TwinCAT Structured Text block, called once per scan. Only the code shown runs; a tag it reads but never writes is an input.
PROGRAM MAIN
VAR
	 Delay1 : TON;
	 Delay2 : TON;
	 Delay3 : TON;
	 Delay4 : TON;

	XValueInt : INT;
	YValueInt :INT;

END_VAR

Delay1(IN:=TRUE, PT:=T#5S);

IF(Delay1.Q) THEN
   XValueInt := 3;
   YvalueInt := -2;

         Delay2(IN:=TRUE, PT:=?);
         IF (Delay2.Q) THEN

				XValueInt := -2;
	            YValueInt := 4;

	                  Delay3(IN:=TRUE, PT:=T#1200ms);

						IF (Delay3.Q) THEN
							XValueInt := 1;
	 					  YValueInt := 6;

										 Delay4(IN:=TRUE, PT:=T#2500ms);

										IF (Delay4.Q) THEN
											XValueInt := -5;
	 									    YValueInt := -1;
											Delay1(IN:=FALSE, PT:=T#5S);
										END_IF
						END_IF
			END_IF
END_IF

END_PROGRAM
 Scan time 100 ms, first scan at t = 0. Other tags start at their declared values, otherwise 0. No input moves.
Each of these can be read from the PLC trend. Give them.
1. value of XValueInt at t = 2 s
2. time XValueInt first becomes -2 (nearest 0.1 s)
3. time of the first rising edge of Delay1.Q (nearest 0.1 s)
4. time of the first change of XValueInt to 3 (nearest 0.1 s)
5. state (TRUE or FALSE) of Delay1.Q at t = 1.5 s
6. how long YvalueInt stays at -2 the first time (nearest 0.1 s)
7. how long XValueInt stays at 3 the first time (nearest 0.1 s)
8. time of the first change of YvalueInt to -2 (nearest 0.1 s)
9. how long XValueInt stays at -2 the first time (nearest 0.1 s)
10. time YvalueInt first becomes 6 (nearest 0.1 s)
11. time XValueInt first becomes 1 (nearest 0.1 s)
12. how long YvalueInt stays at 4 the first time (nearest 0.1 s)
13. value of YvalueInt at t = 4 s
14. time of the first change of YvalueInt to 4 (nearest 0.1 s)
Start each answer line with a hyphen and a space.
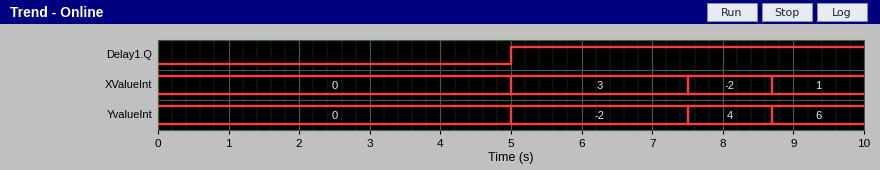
- 0
- 7.5 s
- 5.0 s
- 5.0 s
- FALSE
- 2.5 s
- 2.5 s
- 5.0 s
- 1.2 s
- 8.7 s
- 8.7 s
- 1.2 s
- 0
- 7.5 s
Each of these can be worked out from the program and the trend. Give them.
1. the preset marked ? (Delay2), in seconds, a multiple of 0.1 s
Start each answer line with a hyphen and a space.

- 2.5 s
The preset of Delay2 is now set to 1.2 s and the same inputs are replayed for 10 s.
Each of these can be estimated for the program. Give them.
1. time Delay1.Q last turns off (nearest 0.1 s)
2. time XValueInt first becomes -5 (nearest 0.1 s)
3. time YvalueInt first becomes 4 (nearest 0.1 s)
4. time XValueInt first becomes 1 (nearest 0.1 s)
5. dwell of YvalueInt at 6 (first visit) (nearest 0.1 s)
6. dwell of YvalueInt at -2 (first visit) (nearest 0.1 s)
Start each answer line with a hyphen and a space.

- 9.9 s
- 9.9 s
- 6.2 s
- 7.4 s
- 2.5 s
- 1.2 s
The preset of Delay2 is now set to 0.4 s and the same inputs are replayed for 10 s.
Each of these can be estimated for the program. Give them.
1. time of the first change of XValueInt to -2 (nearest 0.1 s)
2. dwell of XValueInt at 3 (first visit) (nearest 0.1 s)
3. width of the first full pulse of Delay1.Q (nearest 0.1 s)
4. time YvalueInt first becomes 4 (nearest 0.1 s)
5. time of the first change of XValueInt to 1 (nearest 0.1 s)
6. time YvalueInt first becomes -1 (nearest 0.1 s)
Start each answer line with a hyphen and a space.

- 5.4 s
- 0.4 s
- 4.1 s
- 5.4 s
- 6.6 s
- 9.1 s
